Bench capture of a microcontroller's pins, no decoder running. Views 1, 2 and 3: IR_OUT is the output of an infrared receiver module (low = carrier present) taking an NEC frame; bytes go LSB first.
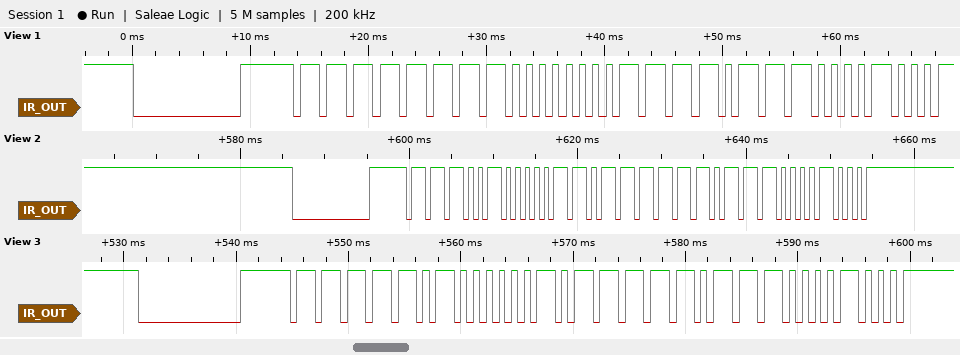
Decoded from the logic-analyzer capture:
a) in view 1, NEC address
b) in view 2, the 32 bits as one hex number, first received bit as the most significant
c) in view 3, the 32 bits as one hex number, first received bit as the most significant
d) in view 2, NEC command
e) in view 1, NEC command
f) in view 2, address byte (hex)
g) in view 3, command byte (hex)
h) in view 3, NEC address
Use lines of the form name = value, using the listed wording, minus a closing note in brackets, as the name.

in view 1, NEC address = 0xFF
in view 2, the 32 bits as one hex number, first received bit as the most significant = 0xE41BF708
in view 3, the 32 bits as one hex number, first received bit as the most significant = 0xFA05F708
in view 2, NEC command = 0xEF
in view 1, NEC command = 0xEF
in view 2, address byte = 0x27
in view 3, command byte = 0xEF
in view 3, NEC address = 0x5F
